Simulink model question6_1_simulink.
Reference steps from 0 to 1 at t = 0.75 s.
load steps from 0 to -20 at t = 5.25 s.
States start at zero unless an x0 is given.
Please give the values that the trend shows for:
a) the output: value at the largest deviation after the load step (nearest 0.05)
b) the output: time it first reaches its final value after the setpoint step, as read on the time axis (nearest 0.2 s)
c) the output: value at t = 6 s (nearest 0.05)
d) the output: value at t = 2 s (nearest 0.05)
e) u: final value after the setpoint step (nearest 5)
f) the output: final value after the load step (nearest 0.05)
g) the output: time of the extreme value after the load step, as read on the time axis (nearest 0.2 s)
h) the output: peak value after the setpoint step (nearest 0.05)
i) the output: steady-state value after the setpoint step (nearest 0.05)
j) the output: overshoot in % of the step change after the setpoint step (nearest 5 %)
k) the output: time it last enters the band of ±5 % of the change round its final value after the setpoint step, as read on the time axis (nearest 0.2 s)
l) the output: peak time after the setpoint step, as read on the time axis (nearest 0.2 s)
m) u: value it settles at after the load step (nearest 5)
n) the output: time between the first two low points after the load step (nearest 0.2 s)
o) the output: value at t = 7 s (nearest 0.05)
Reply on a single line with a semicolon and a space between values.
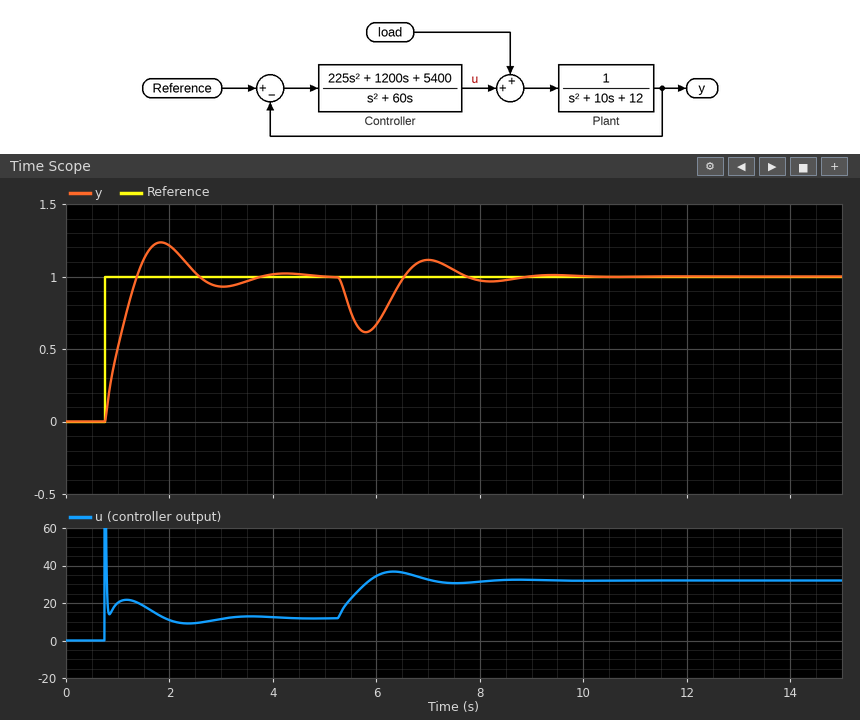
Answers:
0.60; 1.4 s; 0.65; 1.20; 10; 1.00; 5.8 s; 1.25; 1.00; 25 %; 3.4 s; 1.8 s; 30; 2.4 s; 1.10
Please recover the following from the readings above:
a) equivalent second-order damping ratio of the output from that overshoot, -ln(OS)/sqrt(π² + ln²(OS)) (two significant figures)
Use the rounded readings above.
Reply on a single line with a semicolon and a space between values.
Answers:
0.40
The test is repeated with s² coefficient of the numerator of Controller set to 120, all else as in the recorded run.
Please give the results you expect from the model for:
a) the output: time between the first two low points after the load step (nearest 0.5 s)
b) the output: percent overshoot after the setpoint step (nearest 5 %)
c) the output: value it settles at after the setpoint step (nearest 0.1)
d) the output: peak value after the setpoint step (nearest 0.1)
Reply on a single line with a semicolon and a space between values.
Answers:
2.0 s; 30 %; 1.0; 1.3
